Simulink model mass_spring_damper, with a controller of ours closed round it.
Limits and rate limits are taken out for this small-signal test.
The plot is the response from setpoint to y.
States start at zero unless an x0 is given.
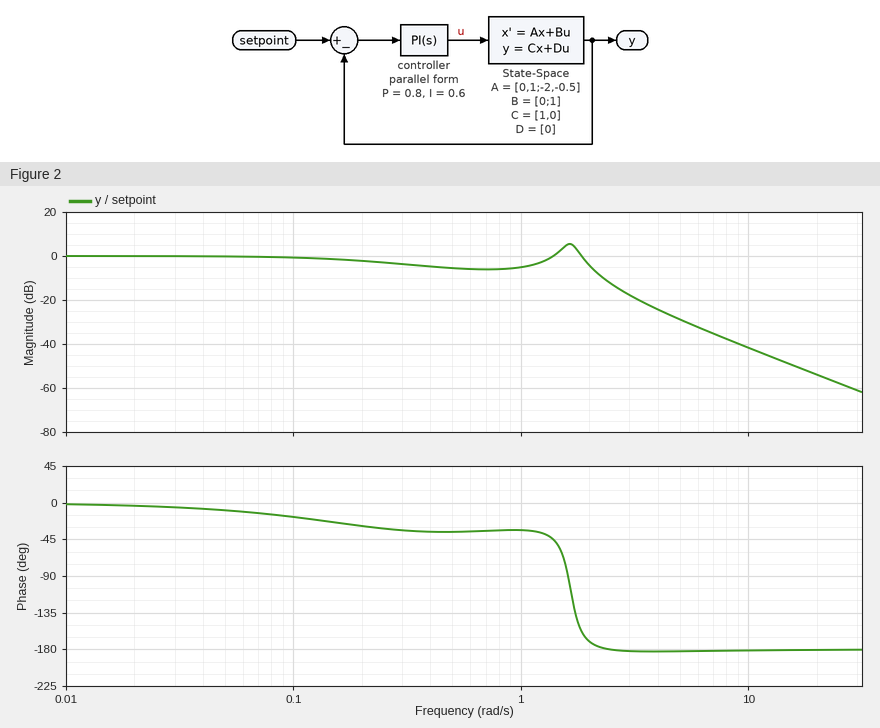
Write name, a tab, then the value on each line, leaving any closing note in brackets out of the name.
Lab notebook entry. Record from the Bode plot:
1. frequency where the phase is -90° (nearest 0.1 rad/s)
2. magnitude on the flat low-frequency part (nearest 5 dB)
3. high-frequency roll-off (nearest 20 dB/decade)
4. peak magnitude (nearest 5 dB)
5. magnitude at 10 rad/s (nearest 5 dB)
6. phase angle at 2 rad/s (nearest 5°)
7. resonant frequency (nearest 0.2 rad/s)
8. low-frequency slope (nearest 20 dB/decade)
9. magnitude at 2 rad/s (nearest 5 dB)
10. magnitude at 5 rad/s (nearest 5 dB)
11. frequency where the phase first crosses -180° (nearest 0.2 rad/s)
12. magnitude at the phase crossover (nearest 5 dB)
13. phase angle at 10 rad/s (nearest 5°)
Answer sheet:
frequency where the phase is -90°	1.6 rad/s
magnitude on the flat low-frequency part	0 dB
high-frequency roll-off	-40 dB/decade
peak magnitude	5 dB
magnitude at 10 rad/s	-40 dB
phase angle at 2 rad/s	-170°
resonant frequency	1.6 rad/s
low-frequency slope	0 dB/decade
magnitude at 2 rad/s	-5 dB
magnitude at 5 rad/s	-30 dB
frequency where the phase first crosses -180°	2.4 rad/s
magnitude at the phase crossover	-10 dB
phase angle at 10 rad/s	-180°
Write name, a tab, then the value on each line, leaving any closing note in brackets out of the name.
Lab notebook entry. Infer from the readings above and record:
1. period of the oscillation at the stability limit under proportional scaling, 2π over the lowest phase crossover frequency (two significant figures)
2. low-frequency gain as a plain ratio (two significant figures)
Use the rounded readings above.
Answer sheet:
period of the oscillation at the stability limit under proportional scaling, 2π over the lowest phase crossover frequency	2.6 s
low-frequency gain as a plain ratio	1.0
